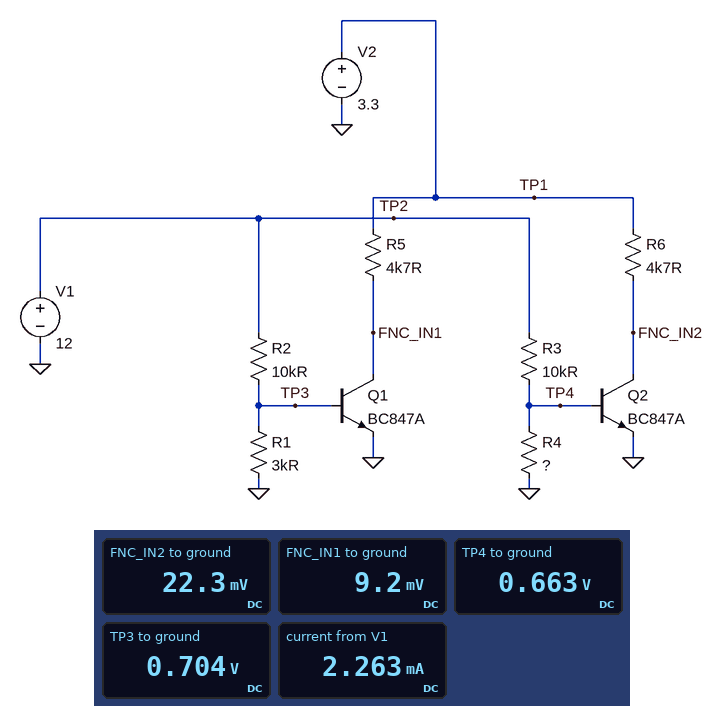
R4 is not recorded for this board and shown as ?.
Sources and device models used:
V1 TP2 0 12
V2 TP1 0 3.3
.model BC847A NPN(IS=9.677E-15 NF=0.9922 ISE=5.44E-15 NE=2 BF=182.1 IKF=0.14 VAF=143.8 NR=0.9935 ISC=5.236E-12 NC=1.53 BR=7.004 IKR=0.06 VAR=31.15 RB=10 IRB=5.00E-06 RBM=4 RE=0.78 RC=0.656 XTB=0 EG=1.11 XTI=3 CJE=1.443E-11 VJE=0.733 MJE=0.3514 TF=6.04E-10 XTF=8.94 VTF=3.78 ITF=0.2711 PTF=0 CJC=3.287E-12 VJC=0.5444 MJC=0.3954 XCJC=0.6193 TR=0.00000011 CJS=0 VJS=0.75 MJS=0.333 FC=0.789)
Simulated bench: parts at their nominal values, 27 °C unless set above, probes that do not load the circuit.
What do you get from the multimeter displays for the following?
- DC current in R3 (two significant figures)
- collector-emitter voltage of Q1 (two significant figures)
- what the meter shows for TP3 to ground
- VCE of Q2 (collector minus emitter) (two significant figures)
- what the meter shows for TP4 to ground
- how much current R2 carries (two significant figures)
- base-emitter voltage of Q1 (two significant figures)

1.1 mA
9.2 mV
0.704 V
22 mV
0.663 V
1.1 mA
700 mV
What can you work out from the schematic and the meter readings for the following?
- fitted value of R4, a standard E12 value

680 Ω
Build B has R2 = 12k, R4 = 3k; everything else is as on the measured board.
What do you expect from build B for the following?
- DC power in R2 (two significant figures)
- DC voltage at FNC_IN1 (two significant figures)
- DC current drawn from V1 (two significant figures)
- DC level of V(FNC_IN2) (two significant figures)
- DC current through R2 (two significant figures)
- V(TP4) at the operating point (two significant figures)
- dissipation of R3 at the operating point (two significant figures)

11 mW
9.9 mV
2.1 mA
9.2 mV
940 µA
700 mV
13 mW
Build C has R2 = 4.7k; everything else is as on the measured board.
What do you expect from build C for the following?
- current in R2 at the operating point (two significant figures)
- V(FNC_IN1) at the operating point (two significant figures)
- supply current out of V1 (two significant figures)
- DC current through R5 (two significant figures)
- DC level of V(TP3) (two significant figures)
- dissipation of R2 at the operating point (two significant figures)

2.4 mA
8.5 mV
3.5 mA
700 µA
730 mV
27 mW
